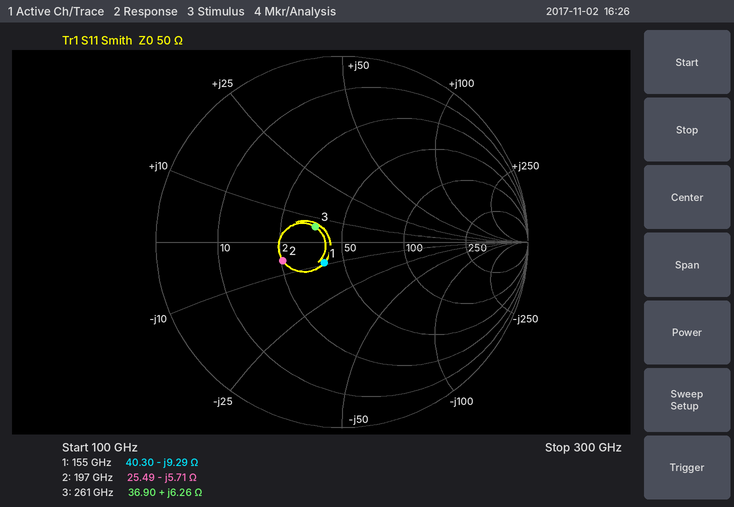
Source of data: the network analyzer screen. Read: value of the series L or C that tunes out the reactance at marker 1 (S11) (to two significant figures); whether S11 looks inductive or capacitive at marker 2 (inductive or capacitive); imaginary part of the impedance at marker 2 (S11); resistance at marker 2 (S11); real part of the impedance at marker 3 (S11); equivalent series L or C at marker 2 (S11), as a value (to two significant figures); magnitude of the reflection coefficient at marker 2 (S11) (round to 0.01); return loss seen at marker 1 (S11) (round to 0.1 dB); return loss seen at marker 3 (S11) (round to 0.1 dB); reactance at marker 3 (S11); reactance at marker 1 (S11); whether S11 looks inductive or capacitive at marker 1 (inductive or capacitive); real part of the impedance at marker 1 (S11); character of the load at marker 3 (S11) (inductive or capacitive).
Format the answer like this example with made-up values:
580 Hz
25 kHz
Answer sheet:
9.5 pH
capacitive
-5.71 Ω
25.49 Ω
36.90 Ω
140 fF
0.33
16.6 dB
15.6 dB
+6.26 Ω
-9.29 Ω
capacitive
40.30 Ω
inductive
